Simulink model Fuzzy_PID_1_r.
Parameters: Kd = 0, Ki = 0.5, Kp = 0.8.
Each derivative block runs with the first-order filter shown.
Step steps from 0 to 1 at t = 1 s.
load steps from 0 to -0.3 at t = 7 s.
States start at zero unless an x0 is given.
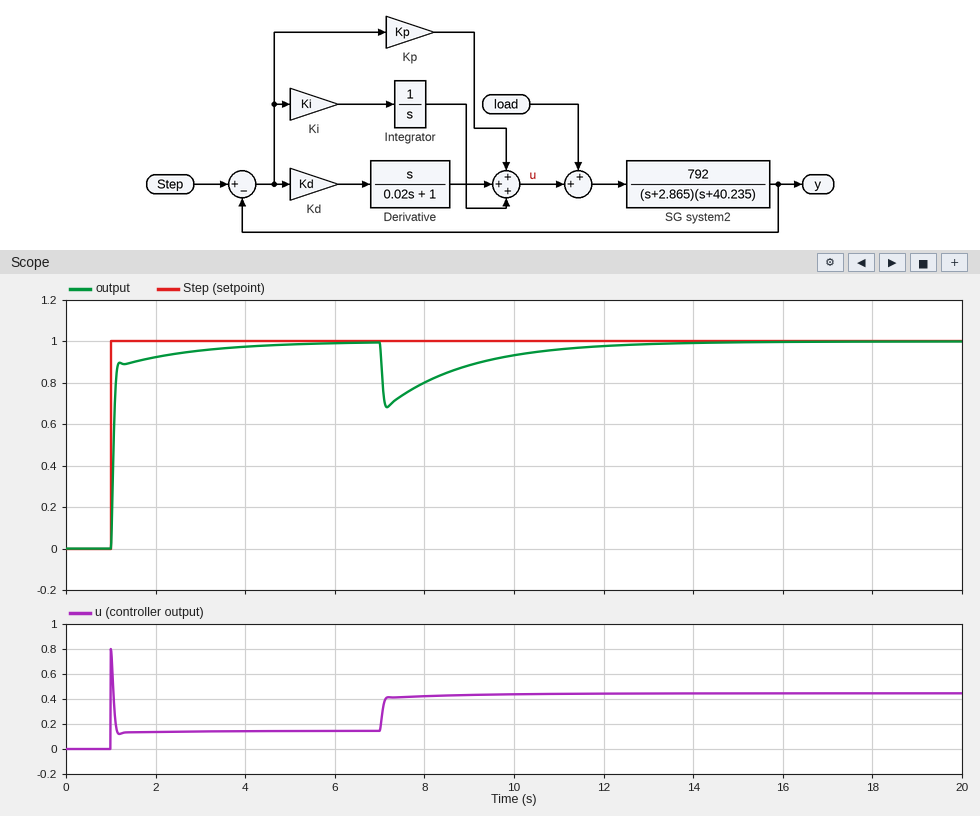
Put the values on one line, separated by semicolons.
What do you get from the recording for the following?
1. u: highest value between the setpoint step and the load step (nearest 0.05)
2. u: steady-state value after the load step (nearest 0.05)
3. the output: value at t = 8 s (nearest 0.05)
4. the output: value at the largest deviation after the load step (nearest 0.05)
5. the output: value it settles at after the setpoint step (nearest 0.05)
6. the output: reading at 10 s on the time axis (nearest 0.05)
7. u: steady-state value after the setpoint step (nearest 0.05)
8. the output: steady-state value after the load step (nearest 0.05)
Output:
0.80; 0.45; 0.80; 0.70; 1.00; 0.95; 0.15; 1.00
